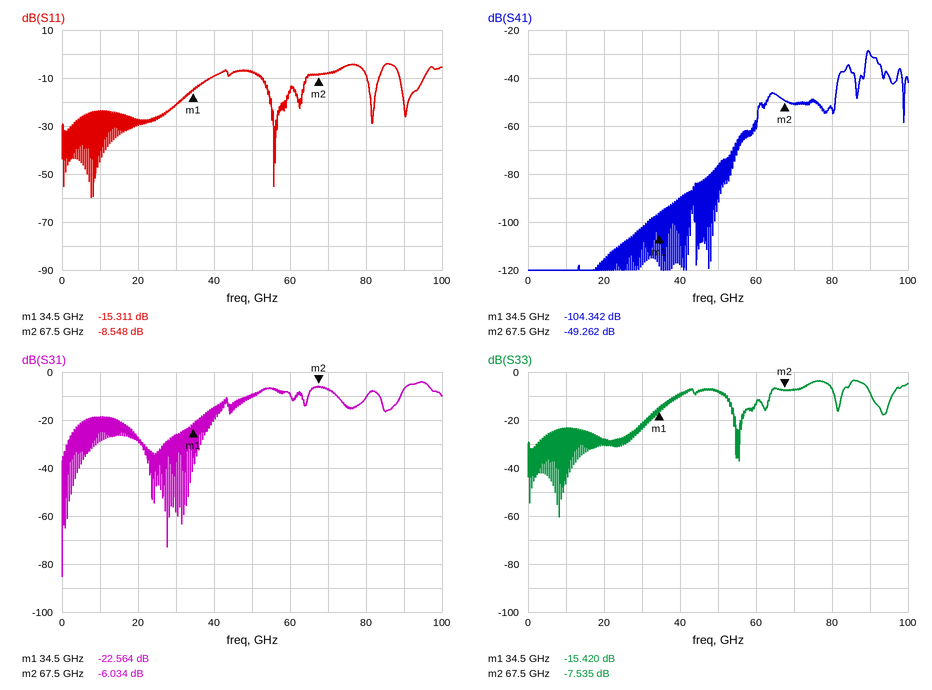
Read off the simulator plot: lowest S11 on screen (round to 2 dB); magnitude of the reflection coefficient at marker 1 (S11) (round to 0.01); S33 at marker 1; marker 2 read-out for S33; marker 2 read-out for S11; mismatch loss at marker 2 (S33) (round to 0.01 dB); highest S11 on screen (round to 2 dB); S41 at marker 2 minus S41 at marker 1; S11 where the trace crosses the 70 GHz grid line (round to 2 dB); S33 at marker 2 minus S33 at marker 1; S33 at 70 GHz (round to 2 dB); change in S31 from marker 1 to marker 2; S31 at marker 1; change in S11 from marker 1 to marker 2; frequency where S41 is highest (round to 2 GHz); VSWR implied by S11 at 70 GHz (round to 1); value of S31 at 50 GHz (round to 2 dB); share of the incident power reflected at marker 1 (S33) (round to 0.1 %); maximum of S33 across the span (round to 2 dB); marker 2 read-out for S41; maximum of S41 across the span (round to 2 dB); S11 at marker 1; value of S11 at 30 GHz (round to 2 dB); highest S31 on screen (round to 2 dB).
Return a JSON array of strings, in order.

["-60 dB", "0.17", "-15.420 dB", "-7.535 dB", "-8.548 dB", "0.84 dB", "-4 dB", "55.080 dB", "-8 dB", "7.885 dB", "-8 dB", "16.530 dB", "-22.564 dB", "6.763 dB", "90 GHz", "2", "-10 dB", "2.9 %", "-4 dB", "-49.262 dB", "-28 dB", "-15.311 dB", "-22 dB", "-4 dB"]
